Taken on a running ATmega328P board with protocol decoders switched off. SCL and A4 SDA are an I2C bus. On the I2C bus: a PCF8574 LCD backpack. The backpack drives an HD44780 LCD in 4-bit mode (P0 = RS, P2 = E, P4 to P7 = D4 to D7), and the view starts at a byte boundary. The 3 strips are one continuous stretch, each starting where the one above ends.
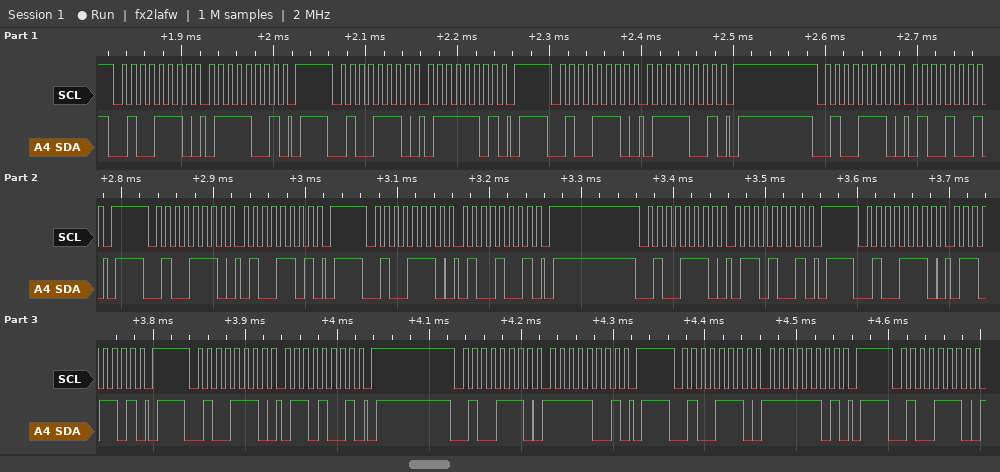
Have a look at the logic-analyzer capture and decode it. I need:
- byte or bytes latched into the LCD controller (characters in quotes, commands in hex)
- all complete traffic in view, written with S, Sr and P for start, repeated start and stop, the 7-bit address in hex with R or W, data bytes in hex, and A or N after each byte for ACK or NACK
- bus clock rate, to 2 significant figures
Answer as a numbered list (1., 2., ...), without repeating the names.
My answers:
1. 't'
2. S 27W A 79 A P S 27W A 7D A P S 27W A 79 A P S 27W A 49 A P S 27W A 4D A P S 27W A 49 A P S 27W A 69 A P S 27W A 6D A P S 27W A 69 A P S 27W A F9 A P S 27W A FD A P S 27W A
3. 100 kHz
